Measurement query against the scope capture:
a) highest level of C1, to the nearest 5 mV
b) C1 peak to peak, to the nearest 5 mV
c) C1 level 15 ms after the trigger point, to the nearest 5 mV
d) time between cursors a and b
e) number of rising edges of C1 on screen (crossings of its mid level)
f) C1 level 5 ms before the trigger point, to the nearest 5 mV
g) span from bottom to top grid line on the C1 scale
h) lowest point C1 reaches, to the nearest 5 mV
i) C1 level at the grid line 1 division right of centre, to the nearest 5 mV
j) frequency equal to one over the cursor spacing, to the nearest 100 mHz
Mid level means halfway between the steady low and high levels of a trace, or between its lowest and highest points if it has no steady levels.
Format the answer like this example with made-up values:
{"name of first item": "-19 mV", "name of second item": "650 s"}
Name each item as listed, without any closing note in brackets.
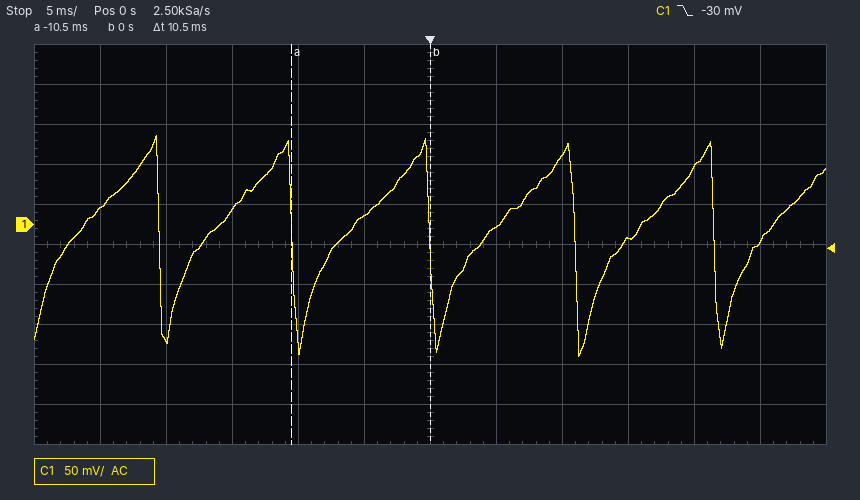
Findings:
{"highest level of C1, to the nearest 5 mV": "110 mV", "C1 peak to peak, to the nearest 5 mV": "275 mV", "C1 level 15 ms after the trigger point, to the nearest 5 mV": "-20 mV", "time between cursors a and b": "10.5 ms", "number of rising edges of C1 on screen": "6", "C1 level 5 ms before the trigger point, to the nearest 5 mV": "10 mV", "span from bottom to top grid line on the C1 scale": "500 mV", "lowest point C1 reaches, to the nearest 5 mV": "-165 mV", "C1 level at the grid line 1 division right of centre, to the nearest 5 mV": "-5 mV", "frequency equal to one over the cursor spacing, to the nearest 100 mHz": "95.2 Hz"}
